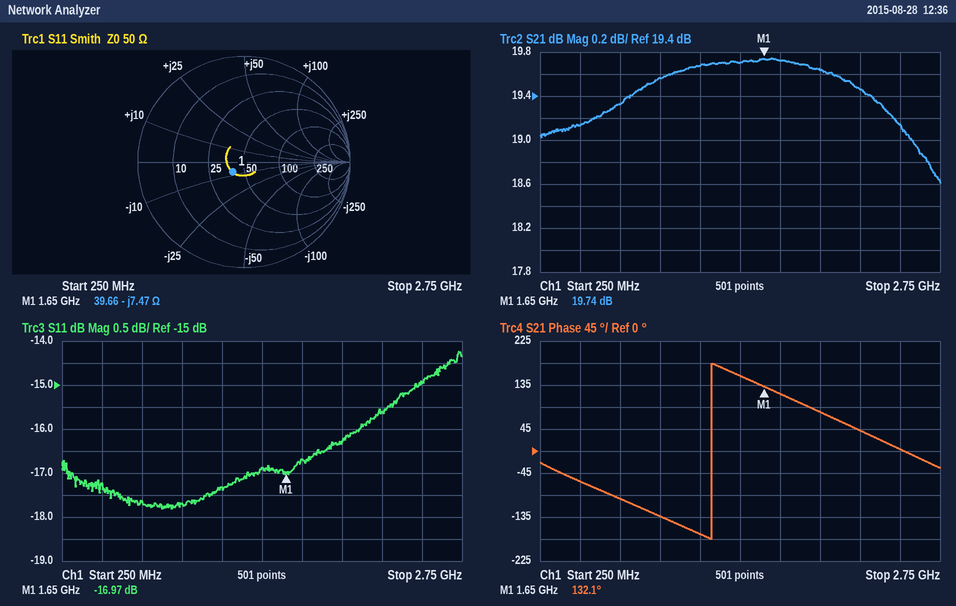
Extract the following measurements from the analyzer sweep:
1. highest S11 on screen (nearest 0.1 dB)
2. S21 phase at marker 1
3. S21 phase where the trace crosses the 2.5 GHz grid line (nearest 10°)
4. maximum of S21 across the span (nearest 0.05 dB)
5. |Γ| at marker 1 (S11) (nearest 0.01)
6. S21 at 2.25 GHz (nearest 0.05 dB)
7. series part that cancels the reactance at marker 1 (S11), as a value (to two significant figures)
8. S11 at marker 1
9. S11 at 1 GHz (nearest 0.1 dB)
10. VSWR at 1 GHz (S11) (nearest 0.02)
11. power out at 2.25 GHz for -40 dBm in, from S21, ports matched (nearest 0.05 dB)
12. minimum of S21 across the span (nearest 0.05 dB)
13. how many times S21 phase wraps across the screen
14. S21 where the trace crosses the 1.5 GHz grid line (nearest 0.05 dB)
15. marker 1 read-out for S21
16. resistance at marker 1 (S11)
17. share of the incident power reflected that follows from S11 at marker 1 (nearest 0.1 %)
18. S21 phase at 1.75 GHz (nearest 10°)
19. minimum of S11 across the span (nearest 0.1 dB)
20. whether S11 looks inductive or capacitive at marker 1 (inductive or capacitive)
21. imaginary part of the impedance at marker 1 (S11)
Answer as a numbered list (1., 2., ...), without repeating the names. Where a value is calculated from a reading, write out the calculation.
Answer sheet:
1. -14.2 dB
2. 132.1°
3. 0°
4. 19.75 dB
5. 0.14
6. 19.45 dB
7. L = 7.47 Ω/(2π × 1.65 GHz) ≈ 721 pH, so 720 pH to two significant figures
8. -16.97 dB
9. -17.7 dB
10. |Γ| = 10^(-17.7/20) = 0.1303; VSWR = (1 + 0.1303)/(1 − 0.1303) ≈ 1.30
11. -40 dBm + (19.45 dB) = -20.55 dBm
12. 18.60 dB
13. 1
14. 19.70 dB
15. 19.74 dB
16. 39.66 Ω
17. 10^(-16.97/10) ≈ 2.0 %
18. 120°
19. -17.8 dB
20. capacitive
21. -7.47 Ω
